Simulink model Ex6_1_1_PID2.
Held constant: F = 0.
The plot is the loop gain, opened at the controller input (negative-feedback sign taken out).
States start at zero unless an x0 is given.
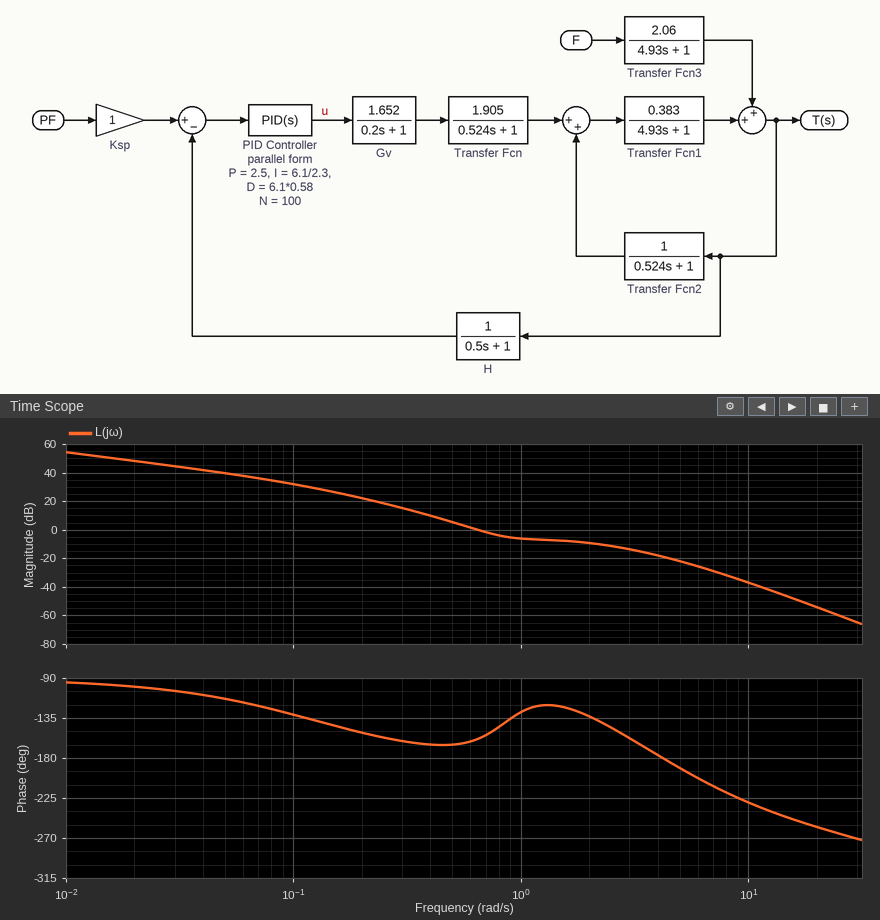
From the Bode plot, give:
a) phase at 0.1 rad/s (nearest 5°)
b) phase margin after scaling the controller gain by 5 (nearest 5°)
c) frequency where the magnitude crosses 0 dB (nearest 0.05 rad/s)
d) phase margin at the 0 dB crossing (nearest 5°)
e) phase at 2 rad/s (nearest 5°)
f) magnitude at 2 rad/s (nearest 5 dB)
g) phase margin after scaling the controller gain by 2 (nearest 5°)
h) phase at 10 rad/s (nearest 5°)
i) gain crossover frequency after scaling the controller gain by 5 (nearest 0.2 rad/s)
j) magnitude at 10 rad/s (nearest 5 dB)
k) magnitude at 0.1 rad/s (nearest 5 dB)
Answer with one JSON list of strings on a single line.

["-130°", "20°", "0.65 rad/s", "20°", "-135°", "-10 dB", "50°", "-230°", "3.0 rad/s", "-35 dB", "30 dB"]
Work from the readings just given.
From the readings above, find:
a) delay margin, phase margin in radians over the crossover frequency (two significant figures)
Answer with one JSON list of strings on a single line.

["0.54 s"]
